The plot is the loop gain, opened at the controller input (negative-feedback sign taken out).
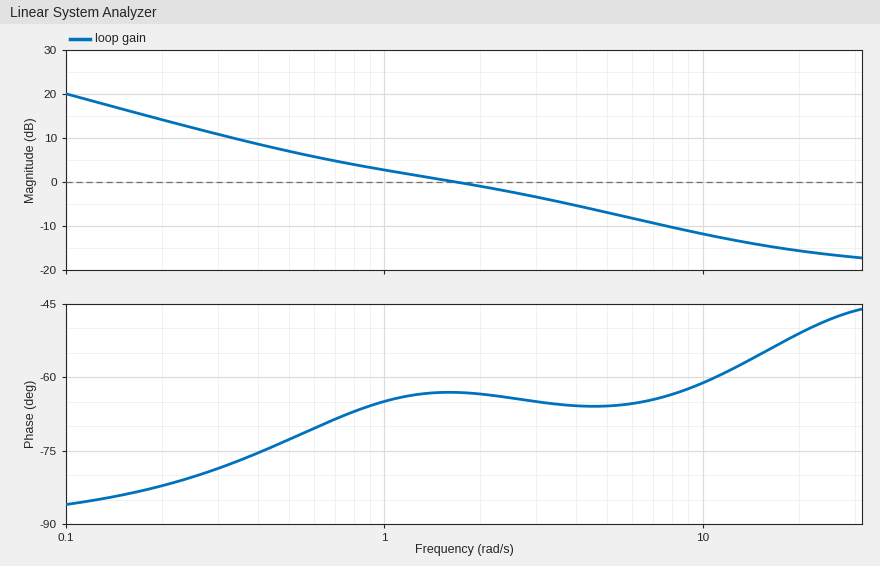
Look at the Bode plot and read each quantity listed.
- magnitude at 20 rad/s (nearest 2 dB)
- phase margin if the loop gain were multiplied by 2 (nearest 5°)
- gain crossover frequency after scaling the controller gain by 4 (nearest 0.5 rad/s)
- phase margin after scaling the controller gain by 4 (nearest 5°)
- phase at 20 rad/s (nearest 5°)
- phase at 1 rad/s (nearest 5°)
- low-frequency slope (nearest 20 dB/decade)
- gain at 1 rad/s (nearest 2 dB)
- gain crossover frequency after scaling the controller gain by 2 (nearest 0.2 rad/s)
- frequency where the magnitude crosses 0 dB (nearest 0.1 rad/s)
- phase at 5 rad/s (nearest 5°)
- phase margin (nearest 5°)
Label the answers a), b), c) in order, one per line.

a) -16 dB
b) 115°
c) 10.5 rad/s
d) 120°
e) -50°
f) -65°
g) -20 dB/decade
h) 2 dB
i) 4.4 rad/s
j) 1.7 rad/s
k) -65°
l) 115°
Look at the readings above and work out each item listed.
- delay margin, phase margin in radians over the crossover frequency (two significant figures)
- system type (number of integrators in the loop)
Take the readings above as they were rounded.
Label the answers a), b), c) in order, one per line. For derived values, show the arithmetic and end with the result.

a) 115 × π / 180 / 1.7 = 1.2 s
b) 1
